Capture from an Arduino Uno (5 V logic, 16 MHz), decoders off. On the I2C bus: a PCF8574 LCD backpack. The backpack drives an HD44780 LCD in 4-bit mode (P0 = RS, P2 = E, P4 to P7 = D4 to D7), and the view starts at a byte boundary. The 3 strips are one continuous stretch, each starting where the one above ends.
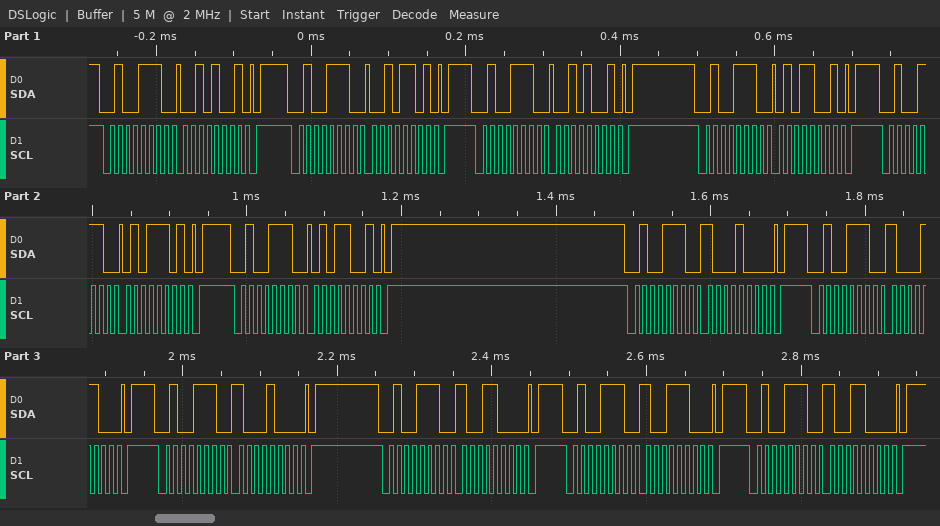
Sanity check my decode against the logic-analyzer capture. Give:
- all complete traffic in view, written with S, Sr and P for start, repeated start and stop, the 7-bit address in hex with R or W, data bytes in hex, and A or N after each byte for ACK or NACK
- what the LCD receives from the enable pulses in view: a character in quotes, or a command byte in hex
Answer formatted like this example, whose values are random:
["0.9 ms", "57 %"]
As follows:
["S 27W A 29 A P S 27W A 2D A P S 27W A 29 A P S 27W A 59 A P S 27W A 5D A P S 27W A 59 A P S 27W A 88 A P S 27W A 8C A P S 27W A 88 A P S 27W A 98 A P S 27W A 9C A P S 27W A 98 A P", "'%' 0x89"]
